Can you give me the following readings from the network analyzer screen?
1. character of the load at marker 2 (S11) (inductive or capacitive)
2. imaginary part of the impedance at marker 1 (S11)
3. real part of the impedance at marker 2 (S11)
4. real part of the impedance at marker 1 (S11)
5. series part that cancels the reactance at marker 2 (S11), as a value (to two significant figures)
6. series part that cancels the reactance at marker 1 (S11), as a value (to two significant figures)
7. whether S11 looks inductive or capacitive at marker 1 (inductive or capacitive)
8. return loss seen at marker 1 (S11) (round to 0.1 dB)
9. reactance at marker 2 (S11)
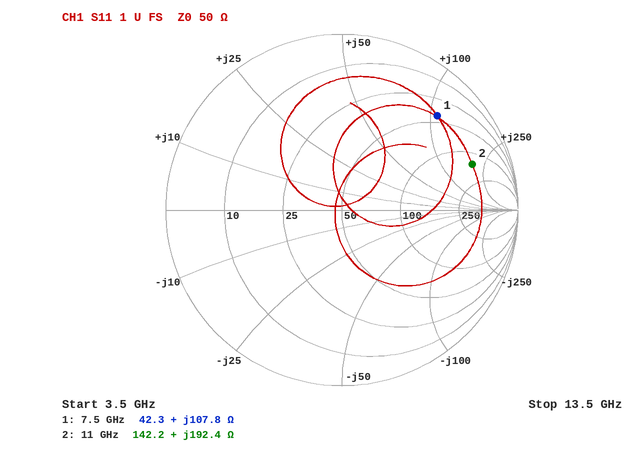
inductive
+107.8 Ω
142.2 Ω
42.3 Ω
75 fF
200 fF
inductive
2.4 dB
+192.4 Ω
